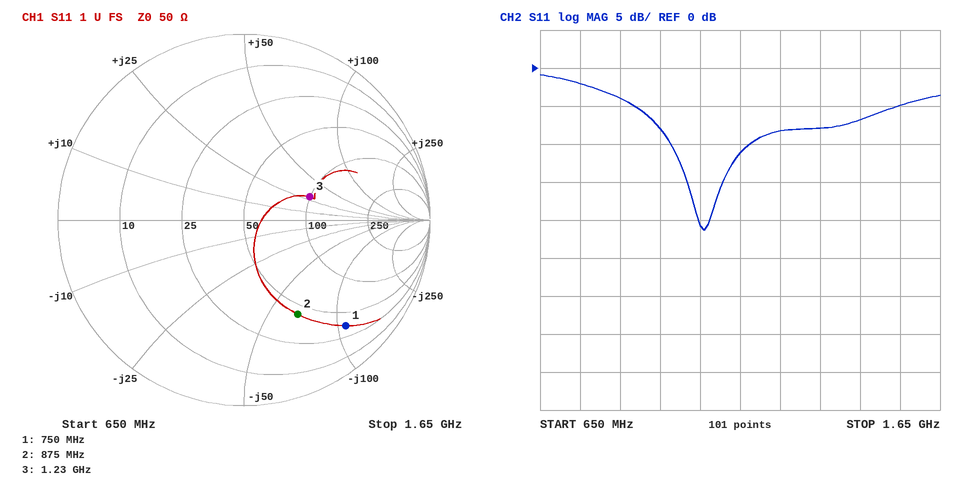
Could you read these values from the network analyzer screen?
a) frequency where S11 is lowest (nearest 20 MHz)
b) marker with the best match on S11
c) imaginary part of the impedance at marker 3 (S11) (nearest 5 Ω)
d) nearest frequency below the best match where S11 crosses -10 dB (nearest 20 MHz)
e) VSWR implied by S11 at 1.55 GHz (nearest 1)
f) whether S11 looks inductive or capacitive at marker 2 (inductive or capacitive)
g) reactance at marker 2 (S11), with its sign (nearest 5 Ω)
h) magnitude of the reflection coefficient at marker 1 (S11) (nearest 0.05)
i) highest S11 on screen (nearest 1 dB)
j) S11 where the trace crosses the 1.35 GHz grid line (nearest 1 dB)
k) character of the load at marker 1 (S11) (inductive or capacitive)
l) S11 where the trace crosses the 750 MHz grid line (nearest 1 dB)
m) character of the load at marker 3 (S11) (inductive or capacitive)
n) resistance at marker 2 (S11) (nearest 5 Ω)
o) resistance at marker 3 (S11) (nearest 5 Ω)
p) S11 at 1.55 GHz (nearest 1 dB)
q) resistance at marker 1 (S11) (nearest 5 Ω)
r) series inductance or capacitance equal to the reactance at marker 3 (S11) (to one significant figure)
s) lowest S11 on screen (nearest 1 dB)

1.06 GHz
marker 3
+30 Ω
980 MHz
4
capacitive
-65 Ω
0.80
-1 dB
-8 dB
capacitive
-2 dB
inductive
45 Ω
100 Ω
-5 dB
35 Ω
4 nH
-21 dB
